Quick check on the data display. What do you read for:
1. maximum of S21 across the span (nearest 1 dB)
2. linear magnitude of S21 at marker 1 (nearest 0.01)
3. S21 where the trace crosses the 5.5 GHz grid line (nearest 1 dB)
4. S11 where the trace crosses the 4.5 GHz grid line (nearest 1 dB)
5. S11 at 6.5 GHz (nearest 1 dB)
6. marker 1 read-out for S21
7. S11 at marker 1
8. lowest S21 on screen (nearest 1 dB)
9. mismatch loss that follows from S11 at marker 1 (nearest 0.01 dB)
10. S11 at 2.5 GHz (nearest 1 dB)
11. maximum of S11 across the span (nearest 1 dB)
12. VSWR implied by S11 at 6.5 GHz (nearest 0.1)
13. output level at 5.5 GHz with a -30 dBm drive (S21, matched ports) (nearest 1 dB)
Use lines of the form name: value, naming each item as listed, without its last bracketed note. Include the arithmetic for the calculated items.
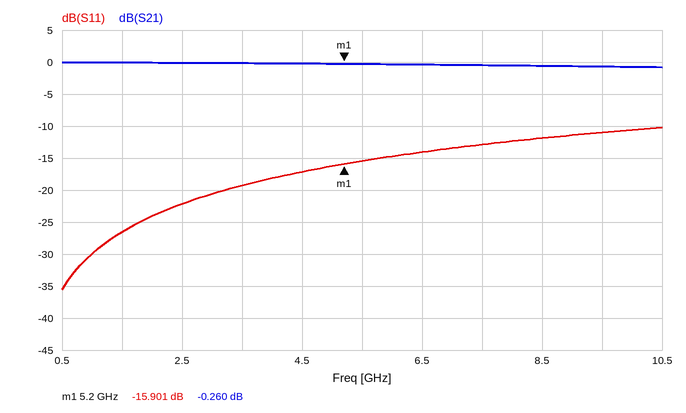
maximum of S21 across the span: 0 dB
linear magnitude of S21 at marker 1: 10^(-0.26/20) ≈ 0.97
S21 where the trace crosses the 5.5 GHz grid line: 0 dB
S11 where the trace crosses the 4.5 GHz grid line: -17 dB
S11 at 6.5 GHz: -14 dB
marker 1 read-out for S21: -0.260 dB
S11 at marker 1: -15.901 dB
lowest S21 on screen: -1 dB
mismatch loss that follows from S11 at marker 1: −10 log10(1 − 10^(-15.901/10)) ≈ 0.11 dB
S11 at 2.5 GHz: -22 dB
maximum of S11 across the span: -10 dB
VSWR implied by S11 at 6.5 GHz: |Γ| = 10^(-14/20) = 0.1995; VSWR = (1 + 0.1995)/(1 − 0.1995) ≈ 1.5
output level at 5.5 GHz with a -30 dBm drive (S21, matched ports): -30 dBm + (0 dB) = -30 dBm
